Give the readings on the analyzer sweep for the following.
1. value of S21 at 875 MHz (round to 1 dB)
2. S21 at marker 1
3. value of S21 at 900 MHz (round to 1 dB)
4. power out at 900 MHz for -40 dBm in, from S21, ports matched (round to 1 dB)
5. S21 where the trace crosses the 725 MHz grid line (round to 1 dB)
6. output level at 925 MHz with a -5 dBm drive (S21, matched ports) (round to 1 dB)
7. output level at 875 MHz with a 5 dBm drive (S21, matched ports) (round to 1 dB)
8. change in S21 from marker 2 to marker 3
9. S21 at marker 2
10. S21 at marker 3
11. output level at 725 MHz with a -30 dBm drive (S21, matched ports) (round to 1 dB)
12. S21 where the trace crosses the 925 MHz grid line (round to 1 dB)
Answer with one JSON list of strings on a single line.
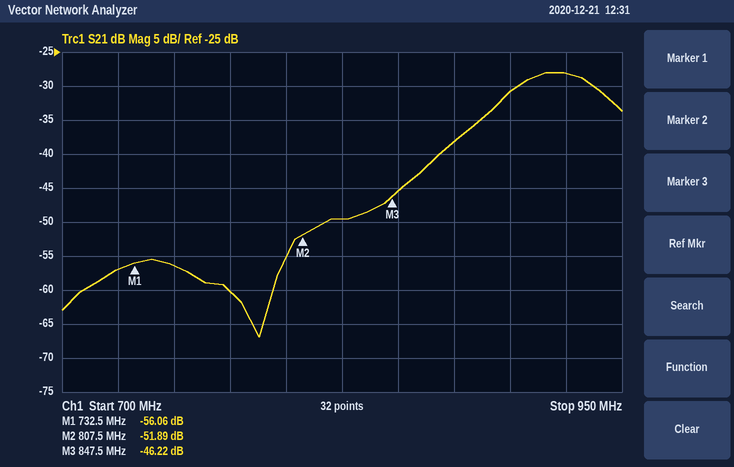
["-38 dB", "-56.06 dB", "-31 dB", "-71 dBm", "-57 dB", "-33 dBm", "-33 dBm", "5.67 dB", "-51.89 dB", "-46.22 dB", "-87 dBm", "-28 dB"]
